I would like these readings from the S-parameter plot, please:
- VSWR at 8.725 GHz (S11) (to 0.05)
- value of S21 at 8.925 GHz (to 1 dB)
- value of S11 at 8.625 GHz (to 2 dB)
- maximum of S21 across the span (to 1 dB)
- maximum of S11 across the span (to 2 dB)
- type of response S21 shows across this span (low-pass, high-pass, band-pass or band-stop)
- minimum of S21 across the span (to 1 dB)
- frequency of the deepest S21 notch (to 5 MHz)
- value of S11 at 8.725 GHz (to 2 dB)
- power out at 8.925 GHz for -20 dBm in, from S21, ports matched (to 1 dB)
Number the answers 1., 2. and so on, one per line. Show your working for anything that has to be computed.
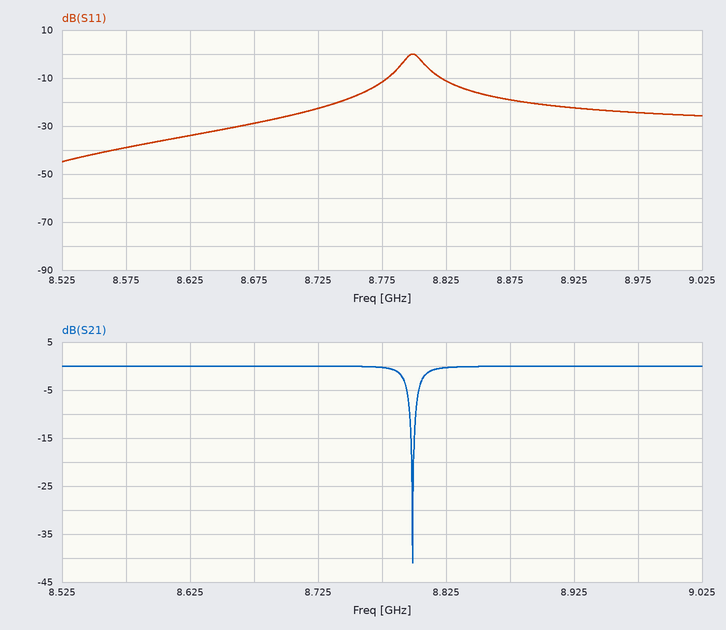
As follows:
1. |Γ| = 10^(-22/20) = 0.0794; VSWR = (1 + 0.0794)/(1 − 0.0794) ≈ 1.17, so 1.15 to the nearest 0.05
2. 0 dB
3. -34 dB
4. 0 dB
5. 0 dB
6. band-stop
7. -41 dB
8. 8.800 GHz
9. -22 dB
10. -20 dBm + (0 dB) = -20 dBm
